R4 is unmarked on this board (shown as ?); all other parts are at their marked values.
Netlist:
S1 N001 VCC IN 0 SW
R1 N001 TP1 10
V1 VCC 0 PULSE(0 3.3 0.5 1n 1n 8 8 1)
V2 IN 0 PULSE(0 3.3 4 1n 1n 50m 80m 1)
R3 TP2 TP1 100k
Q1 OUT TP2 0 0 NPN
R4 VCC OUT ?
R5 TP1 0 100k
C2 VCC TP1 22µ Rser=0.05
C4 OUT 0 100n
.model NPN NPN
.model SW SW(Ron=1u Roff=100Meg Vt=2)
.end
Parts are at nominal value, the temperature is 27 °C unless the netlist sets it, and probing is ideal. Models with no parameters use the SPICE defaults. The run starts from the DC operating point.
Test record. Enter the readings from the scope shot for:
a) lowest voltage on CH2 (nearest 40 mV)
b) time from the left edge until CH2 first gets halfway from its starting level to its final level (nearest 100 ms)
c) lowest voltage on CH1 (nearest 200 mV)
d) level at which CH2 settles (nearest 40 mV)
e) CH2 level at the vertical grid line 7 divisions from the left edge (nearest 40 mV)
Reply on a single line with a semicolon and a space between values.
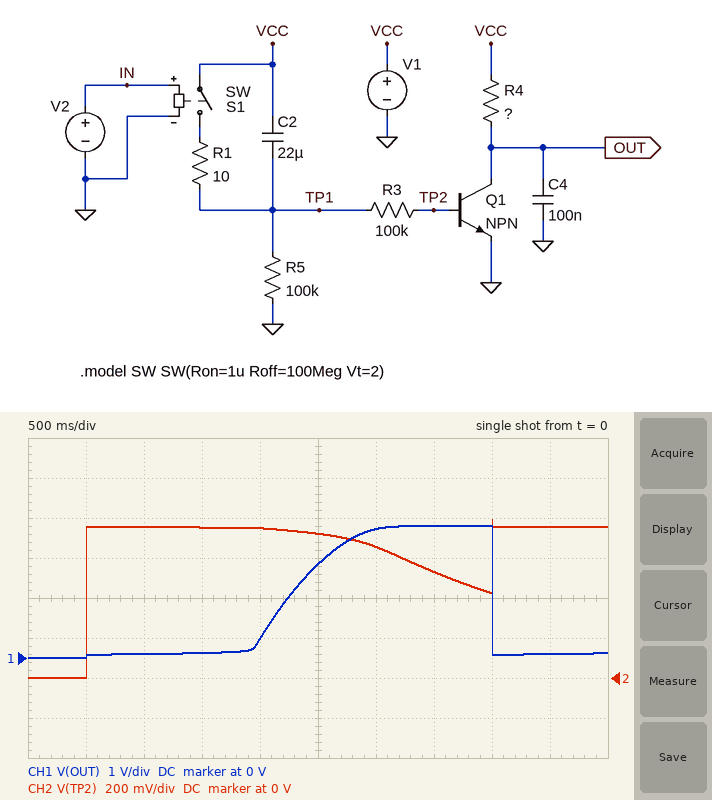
0 V; 500 ms; 0 V; 760 mV; 520 mV
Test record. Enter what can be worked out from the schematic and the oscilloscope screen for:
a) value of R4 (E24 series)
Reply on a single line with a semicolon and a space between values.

7.5 kΩ
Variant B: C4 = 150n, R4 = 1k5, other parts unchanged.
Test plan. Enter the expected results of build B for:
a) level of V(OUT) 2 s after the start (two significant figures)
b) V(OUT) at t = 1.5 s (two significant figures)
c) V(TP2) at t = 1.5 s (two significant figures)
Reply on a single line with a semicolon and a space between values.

2.7 V; 2.1 V; 770 mV
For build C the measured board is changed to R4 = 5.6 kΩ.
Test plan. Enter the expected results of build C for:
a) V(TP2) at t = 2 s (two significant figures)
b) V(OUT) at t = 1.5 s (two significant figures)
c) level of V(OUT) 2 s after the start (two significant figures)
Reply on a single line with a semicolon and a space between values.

750 mV; 140 mV; 1.2 V
